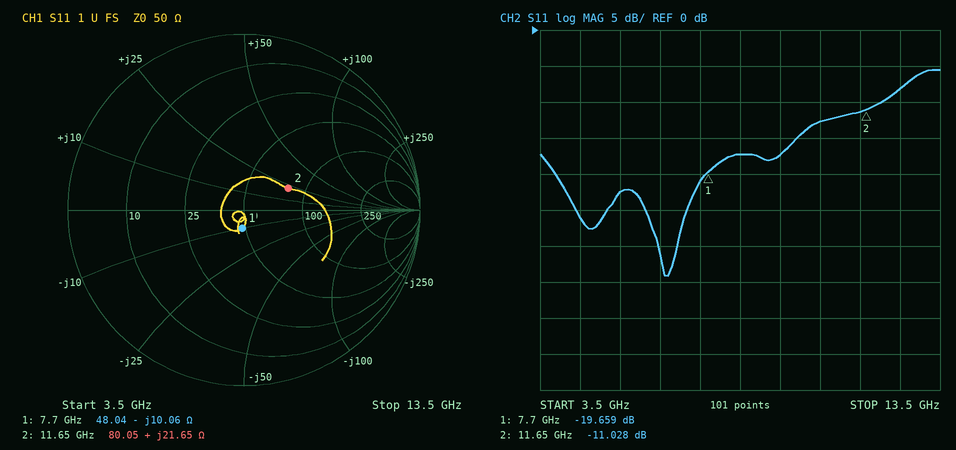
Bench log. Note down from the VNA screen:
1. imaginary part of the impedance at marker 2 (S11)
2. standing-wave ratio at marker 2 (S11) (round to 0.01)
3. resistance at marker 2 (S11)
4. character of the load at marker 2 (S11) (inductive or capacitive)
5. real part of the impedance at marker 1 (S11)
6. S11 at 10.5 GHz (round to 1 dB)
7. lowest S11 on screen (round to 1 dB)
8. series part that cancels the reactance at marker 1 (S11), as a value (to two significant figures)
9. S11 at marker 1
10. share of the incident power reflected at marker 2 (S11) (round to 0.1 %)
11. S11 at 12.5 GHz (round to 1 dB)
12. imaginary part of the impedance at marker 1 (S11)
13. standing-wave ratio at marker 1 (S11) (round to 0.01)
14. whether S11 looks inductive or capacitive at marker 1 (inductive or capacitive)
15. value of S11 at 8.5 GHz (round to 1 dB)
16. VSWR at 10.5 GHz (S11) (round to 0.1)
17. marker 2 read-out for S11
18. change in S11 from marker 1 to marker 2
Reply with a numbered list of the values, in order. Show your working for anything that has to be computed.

1. +21.65 Ω
2. 1.78
3. 80.05 Ω
4. inductive
5. 48.04 Ω
6. -13 dB
7. -34 dB
8. L = 10.06 Ω/(2π × 7.7 GHz) ≈ 208 pH, so 210 pH to two significant figures
9. -19.659 dB
10. 10^(-11.028/10) ≈ 7.9 %
11. -8 dB
12. -10.06 Ω
13. 1.23
14. capacitive
15. -17 dB
16. |Γ| = 10^(-13/20) = 0.2239; VSWR = (1 + 0.2239)/(1 − 0.2239) ≈ 1.6
17. -11.028 dB
18. -11.028 − (-19.659) = 8.631 dB
